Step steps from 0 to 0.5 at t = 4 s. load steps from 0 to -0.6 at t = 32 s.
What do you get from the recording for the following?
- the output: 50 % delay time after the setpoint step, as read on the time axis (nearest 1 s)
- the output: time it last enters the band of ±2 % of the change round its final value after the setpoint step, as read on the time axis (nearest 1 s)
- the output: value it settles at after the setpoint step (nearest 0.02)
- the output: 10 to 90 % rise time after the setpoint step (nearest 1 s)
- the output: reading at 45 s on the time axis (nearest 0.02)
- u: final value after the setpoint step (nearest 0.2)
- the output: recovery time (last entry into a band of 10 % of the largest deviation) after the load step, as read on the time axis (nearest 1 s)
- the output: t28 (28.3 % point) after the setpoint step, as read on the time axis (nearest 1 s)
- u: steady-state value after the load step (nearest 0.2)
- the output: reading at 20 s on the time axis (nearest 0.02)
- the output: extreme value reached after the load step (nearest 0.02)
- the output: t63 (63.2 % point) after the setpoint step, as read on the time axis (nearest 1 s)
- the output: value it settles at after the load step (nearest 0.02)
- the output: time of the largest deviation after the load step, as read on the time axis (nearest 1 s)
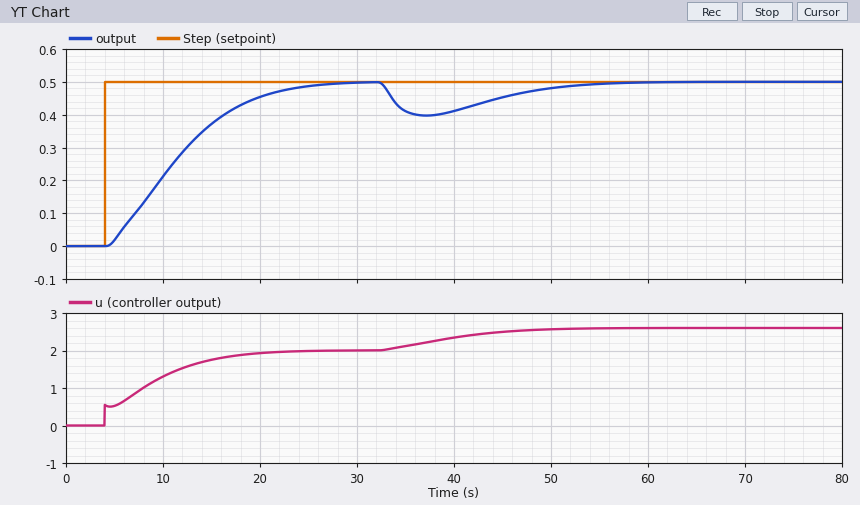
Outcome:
11 s
26 s
0.50
14 s
0.46
2.0
53 s
8 s
2.6
0.46
0.40
13 s
0.50
37 s
